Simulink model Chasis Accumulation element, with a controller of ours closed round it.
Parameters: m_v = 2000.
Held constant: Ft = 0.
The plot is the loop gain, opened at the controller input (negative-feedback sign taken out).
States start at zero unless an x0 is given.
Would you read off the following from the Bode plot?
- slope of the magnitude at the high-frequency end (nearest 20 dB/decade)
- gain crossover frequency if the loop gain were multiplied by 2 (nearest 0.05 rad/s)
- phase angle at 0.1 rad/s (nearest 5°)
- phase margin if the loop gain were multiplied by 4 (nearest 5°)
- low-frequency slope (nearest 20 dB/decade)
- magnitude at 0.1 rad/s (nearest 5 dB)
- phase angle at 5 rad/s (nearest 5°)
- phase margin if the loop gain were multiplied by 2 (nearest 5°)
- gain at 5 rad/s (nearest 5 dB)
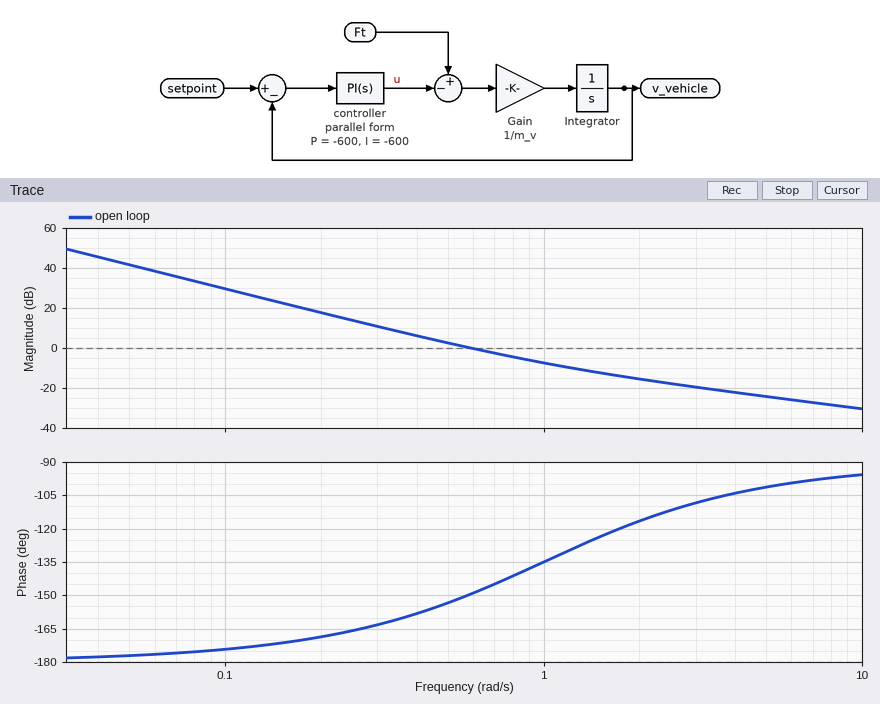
-20 dB/decade
0.90 rad/s
-175°
55°
-40 dB/decade
30 dB
-100°
40°
-25 dB
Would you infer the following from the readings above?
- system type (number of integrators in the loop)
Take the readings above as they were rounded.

2
